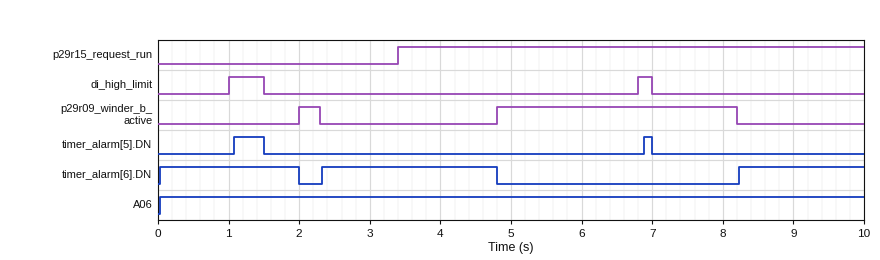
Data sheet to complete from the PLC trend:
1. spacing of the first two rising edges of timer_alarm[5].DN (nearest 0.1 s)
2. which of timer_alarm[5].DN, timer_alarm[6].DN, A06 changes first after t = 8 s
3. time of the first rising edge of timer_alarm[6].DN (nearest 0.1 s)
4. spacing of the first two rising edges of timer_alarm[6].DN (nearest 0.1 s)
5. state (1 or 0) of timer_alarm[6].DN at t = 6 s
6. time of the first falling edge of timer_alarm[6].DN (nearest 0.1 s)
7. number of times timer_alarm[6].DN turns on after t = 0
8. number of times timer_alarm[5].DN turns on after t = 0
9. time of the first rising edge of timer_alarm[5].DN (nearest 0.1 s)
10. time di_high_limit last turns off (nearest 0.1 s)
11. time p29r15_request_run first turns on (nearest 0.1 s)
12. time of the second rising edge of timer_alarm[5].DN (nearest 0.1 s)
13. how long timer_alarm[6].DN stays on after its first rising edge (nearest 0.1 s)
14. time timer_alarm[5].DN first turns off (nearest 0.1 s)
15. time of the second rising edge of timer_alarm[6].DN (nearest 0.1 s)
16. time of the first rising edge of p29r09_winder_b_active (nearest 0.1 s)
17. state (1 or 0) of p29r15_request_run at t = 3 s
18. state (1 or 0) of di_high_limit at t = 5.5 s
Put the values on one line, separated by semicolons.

5.8 s; timer_alarm[6].DN; 0.0 s; 2.3 s; 0; 2.0 s; 3; 2; 1.1 s; 7.0 s; 3.4 s; 6.9 s; 2.0 s; 1.5 s; 2.3 s; 2.0 s; 0; 0
